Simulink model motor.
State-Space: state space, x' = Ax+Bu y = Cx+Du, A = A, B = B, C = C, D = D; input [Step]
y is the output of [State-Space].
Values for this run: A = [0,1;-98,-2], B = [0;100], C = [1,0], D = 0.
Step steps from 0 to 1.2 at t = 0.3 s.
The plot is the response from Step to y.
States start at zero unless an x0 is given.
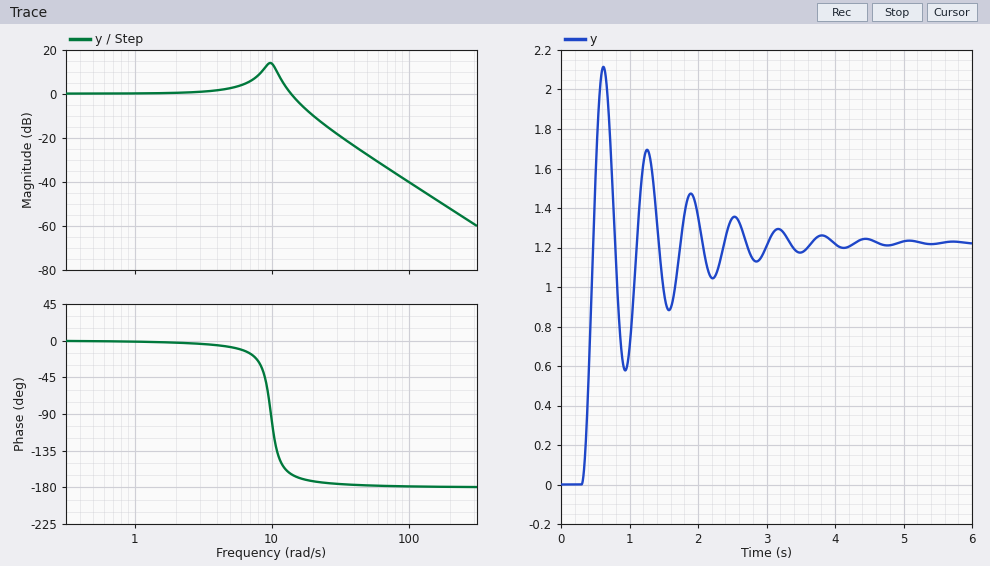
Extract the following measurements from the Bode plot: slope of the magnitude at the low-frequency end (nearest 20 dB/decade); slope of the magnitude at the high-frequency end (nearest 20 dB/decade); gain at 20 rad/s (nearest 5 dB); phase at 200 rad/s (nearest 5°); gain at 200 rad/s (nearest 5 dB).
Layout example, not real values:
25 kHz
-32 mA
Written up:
0 dB/decade
-40 dB/decade
-10 dB
-180°
-50 dB
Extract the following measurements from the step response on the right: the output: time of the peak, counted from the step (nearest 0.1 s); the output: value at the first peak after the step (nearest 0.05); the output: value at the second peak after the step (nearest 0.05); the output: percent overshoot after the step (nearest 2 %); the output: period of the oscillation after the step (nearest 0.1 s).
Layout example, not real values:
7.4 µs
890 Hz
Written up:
0.3 s
2.10
1.70
72 %
0.6 s
